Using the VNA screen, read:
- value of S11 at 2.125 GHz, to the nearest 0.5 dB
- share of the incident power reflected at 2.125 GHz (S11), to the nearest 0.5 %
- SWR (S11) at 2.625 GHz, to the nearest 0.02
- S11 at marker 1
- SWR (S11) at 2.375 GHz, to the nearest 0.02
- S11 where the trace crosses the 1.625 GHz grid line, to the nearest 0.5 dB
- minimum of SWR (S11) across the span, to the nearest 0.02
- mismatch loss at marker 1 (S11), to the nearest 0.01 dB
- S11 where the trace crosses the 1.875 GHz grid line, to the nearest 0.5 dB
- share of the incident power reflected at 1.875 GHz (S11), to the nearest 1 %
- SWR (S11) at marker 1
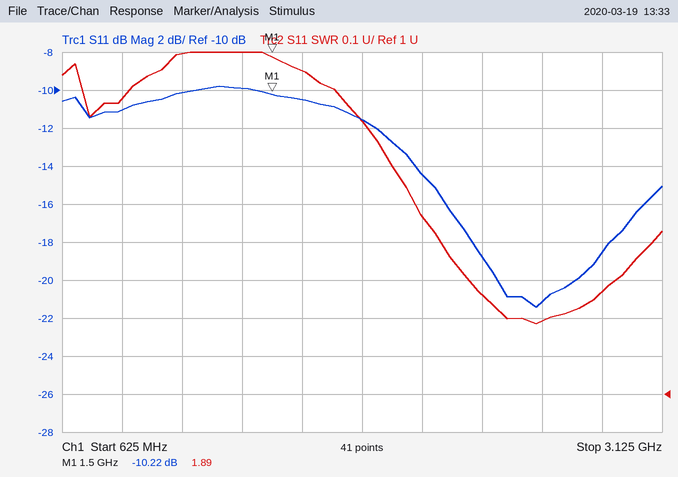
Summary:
-14.5 dB
3.5 %
1.20
-10.22 dB
1.26
-10.5 dB
1.18
0.43 dB
-11.5 dB
7 %
1.89
